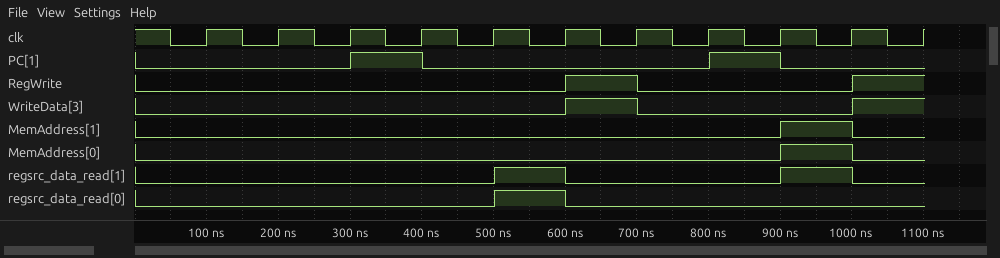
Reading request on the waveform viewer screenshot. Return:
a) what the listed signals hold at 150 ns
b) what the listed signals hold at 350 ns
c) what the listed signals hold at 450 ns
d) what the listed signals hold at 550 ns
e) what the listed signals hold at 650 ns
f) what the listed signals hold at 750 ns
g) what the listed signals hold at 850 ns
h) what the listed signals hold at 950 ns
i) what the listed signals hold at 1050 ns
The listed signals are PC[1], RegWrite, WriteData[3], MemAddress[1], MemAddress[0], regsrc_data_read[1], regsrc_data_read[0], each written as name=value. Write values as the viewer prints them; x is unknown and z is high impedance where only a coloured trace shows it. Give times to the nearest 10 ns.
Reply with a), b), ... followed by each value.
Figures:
a) PC[1]=0, RegWrite=0, WriteData[3]=0, MemAddress[1]=0, MemAddress[0]=0, regsrc_data_read[1]=0, regsrc_data_read[0]=0
b) PC[1]=1, RegWrite=0, WriteData[3]=0, MemAddress[1]=0, MemAddress[0]=0, regsrc_data_read[1]=0, regsrc_data_read[0]=0
c) PC[1]=0, RegWrite=0, WriteData[3]=0, MemAddress[1]=0, MemAddress[0]=0, regsrc_data_read[1]=0, regsrc_data_read[0]=0
d) PC[1]=0, RegWrite=0, WriteData[3]=0, MemAddress[1]=0, MemAddress[0]=0, regsrc_data_read[1]=1, regsrc_data_read[0]=1
e) PC[1]=0, RegWrite=1, WriteData[3]=1, MemAddress[1]=0, MemAddress[0]=0, regsrc_data_read[1]=0, regsrc_data_read[0]=0
f) PC[1]=0, RegWrite=0, WriteData[3]=0, MemAddress[1]=0, MemAddress[0]=0, regsrc_data_read[1]=0, regsrc_data_read[0]=0
g) PC[1]=1, RegWrite=0, WriteData[3]=0, MemAddress[1]=0, MemAddress[0]=0, regsrc_data_read[1]=0, regsrc_data_read[0]=0
h) PC[1]=0, RegWrite=0, WriteData[3]=0, MemAddress[1]=1, MemAddress[0]=1, regsrc_data_read[1]=1, regsrc_data_read[0]=0
i) PC[1]=0, RegWrite=1, WriteData[3]=1, MemAddress[1]=0, MemAddress[0]=0, regsrc_data_read[1]=0, regsrc_data_read[0]=0
